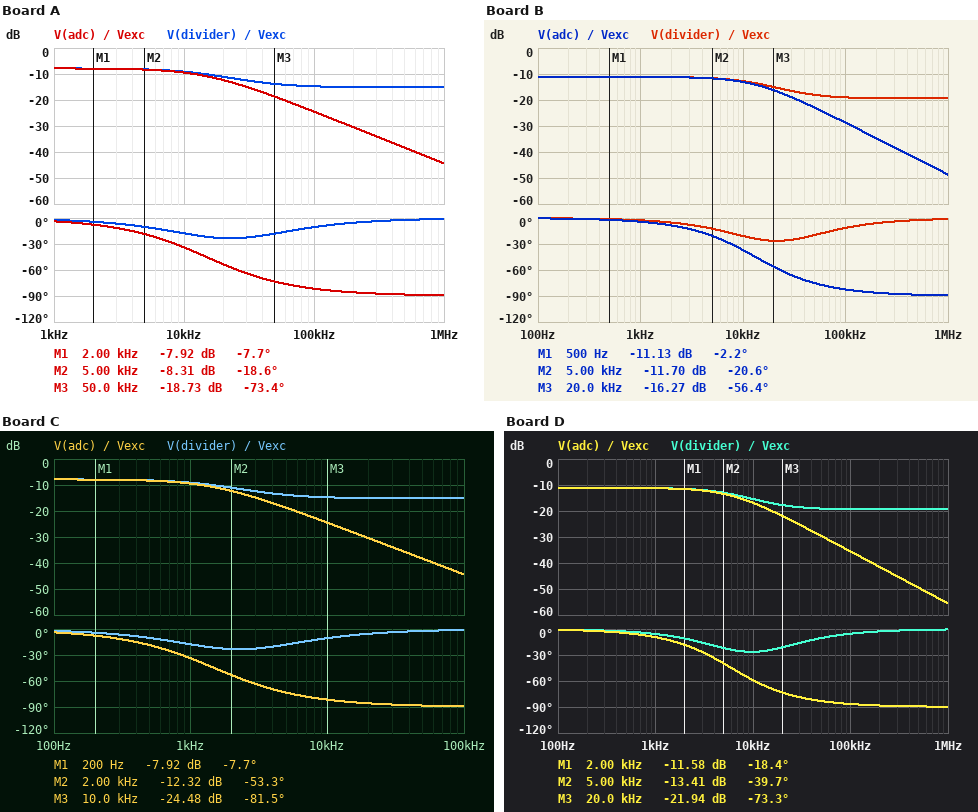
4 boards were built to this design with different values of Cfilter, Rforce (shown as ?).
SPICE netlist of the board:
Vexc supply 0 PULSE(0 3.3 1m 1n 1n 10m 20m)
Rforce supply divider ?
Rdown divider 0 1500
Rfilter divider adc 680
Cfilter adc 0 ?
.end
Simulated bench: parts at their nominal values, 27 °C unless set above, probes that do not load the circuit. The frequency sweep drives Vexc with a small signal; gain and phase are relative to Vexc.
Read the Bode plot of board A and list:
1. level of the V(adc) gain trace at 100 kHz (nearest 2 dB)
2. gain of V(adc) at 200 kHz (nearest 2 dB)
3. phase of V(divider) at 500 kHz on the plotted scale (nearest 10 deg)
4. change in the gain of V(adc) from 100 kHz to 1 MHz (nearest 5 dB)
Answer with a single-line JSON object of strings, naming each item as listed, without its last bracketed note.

{"level of the V(adc) gain trace at 100 kHz": "-24 dB", "gain of V(adc) at 200 kHz": "-30 dB", "phase of V(divider) at 500 kHz on the plotted scale": "0 deg", "change in the gain of V(adc) from 100 kHz to 1 MHz": "-20 dB"}
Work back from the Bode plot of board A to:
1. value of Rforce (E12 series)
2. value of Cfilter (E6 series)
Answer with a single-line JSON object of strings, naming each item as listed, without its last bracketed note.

{"value of Rforce": "2.2 kΩ", "value of Cfilter": "6.8 nF"}
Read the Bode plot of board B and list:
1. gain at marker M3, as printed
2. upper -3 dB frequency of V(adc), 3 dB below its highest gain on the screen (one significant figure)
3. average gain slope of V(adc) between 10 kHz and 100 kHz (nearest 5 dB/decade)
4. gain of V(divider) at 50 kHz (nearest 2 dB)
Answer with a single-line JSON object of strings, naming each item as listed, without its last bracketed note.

{"gain at marker M3, as printed": "-16.27 dB", "upper -3 dB frequency of V(adc), 3 dB below its highest gain on the screen": "10 kHz", "average gain slope of V(adc) between 10 kHz and 100 kHz": "-15 dB/decade", "gain of V(divider) at 50 kHz": "-18 dB"}
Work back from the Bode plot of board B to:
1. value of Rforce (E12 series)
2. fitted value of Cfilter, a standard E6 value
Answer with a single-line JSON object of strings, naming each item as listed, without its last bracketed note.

{"value of Rforce": "3.9 kΩ", "fitted value of Cfilter, a standard E6 value": "6.8 nF"}
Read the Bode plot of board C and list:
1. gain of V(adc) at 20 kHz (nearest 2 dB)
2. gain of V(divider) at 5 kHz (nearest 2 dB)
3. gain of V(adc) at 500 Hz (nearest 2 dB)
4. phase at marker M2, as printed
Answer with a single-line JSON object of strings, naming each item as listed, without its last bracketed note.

{"gain of V(adc) at 20 kHz": "-30 dB", "gain of V(divider) at 5 kHz": "-14 dB", "gain of V(adc) at 500 Hz": "-8 dB", "phase at marker M2, as printed": "-53.3 deg"}
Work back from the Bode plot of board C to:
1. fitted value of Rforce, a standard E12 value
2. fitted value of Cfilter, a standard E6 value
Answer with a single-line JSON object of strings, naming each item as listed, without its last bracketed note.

{"fitted value of Rforce, a standard E12 value": "2.2 kΩ", "fitted value of Cfilter, a standard E6 value": "68 nF"}
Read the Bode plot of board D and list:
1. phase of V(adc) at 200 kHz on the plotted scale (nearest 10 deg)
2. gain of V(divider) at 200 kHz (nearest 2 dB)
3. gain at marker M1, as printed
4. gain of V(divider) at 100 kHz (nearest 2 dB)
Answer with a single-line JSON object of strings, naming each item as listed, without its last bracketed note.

{"phase of V(adc) at 200 kHz on the plotted scale": "-90 deg", "gain of V(divider) at 200 kHz": "-20 dB", "gain at marker M1, as printed": "-11.58 dB", "gain of V(divider) at 100 kHz": "-20 dB"}
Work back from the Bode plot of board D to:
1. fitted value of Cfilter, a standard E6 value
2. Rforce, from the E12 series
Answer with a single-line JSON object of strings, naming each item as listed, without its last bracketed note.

{"fitted value of Cfilter, a standard E6 value": "15 nF", "Rforce, from the E12 series": "3.9 kΩ"}
